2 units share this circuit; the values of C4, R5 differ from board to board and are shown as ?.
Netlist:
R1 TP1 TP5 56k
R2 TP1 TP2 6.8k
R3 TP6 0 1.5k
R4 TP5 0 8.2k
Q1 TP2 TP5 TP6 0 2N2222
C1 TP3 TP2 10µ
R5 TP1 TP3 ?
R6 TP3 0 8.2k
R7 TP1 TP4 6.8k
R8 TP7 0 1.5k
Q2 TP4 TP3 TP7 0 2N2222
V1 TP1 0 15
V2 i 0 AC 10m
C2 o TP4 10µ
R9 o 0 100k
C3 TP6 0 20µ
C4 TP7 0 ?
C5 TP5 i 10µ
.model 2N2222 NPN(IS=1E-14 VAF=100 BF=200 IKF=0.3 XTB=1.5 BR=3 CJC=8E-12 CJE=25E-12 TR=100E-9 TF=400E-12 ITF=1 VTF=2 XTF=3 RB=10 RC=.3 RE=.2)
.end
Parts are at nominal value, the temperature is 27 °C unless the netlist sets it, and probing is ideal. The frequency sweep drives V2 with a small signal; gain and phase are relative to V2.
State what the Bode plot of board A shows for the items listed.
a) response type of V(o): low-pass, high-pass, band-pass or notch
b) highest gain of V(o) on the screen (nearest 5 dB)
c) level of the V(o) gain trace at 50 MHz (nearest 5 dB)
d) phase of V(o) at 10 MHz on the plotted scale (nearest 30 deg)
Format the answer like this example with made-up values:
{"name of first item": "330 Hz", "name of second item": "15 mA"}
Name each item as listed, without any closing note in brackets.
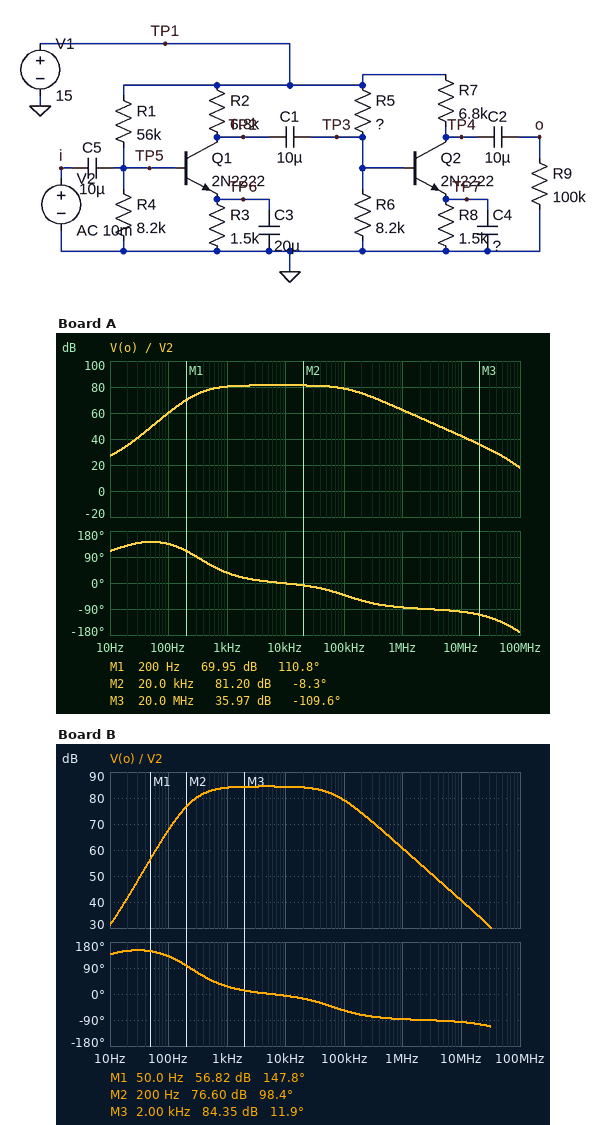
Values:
{"response type of V(o): low-pass, high-pass, band-pass or notch": "band-pass", "highest gain of V(o) on the screen": "80 dB", "level of the V(o) gain trace at 50 MHz": "25 dB", "phase of V(o) at 10 MHz on the plotted scale": "-90 deg"}
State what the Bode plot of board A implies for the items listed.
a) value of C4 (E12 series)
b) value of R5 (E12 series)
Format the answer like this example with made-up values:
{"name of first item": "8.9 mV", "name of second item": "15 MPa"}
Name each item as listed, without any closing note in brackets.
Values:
{"value of C4": "6.8 µF", "value of R5": "68 kΩ"}
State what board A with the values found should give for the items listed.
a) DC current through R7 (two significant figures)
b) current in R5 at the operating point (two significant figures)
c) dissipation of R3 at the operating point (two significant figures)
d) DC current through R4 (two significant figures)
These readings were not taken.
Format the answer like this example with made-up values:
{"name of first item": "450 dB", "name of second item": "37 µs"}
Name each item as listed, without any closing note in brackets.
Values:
{"DC current through R7": "630 µA", "current in R5 at the operating point": "200 µA", "dissipation of R3 at the operating point": "1.0 mW", "DC current through R4": "230 µA"}
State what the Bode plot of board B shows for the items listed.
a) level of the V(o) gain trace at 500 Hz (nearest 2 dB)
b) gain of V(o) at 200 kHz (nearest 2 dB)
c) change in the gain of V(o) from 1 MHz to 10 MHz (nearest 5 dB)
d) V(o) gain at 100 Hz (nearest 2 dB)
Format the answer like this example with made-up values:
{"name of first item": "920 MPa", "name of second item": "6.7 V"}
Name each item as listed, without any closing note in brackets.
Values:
{"level of the V(o) gain trace at 500 Hz": "82 dB", "gain of V(o) at 200 kHz": "74 dB", "change in the gain of V(o) from 1 MHz to 10 MHz": "-20 dB", "V(o) gain at 100 Hz": "68 dB"}
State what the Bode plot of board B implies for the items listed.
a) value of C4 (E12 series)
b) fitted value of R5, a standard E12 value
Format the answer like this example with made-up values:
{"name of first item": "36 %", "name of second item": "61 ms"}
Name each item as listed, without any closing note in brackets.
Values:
{"value of C4": "18 µF", "fitted value of R5, a standard E12 value": "39 kΩ"}
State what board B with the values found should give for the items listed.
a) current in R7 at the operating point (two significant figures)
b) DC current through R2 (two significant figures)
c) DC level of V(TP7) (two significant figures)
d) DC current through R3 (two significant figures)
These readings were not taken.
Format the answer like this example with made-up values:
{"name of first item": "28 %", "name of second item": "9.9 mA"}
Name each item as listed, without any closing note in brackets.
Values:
{"current in R7 at the operating point": "1.3 mA", "DC current through R2": "820 µA", "DC level of V(TP7)": "1.9 V", "DC current through R3": "830 µA"}
